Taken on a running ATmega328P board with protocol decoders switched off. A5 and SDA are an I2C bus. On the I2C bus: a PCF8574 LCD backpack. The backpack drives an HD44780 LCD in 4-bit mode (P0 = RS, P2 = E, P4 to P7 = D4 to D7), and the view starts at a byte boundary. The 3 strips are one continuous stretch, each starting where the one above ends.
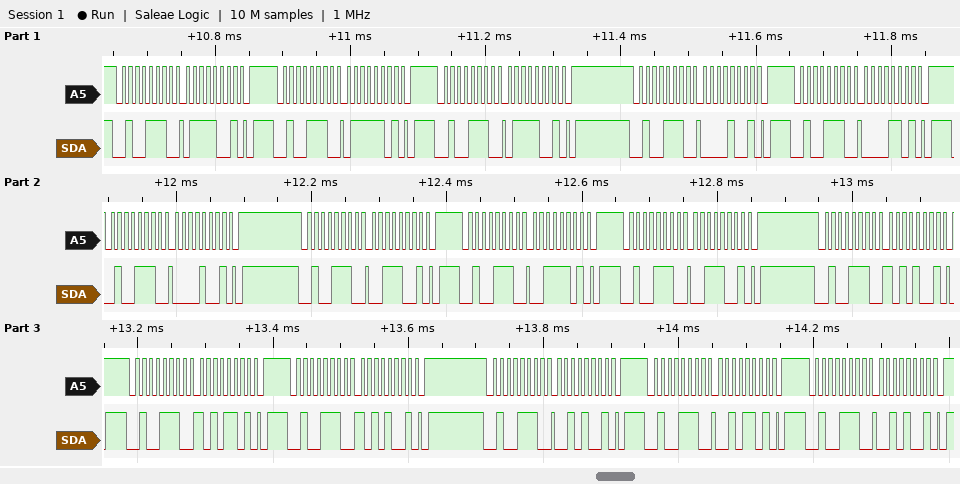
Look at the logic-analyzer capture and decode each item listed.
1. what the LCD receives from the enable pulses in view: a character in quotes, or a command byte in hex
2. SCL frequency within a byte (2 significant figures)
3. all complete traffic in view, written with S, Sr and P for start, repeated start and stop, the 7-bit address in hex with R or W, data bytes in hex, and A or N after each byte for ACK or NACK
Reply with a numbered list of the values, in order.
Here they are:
1. 'p' ':'
2. 100 kHz
3. S 27W A 79 A P S 27W A 7D A P S 27W A 79 A P S 27W A 09 A P S 27W A 0D A P S 27W A 09 A P S 27W A 39 A P S 27W A 3D A P S 27W A 39 A P S 27W A A9 A P S 27W A AD A P S 27W A A9 A P S 27W A 29 A P S 27W A 2D A P S 27W A 29 A P
